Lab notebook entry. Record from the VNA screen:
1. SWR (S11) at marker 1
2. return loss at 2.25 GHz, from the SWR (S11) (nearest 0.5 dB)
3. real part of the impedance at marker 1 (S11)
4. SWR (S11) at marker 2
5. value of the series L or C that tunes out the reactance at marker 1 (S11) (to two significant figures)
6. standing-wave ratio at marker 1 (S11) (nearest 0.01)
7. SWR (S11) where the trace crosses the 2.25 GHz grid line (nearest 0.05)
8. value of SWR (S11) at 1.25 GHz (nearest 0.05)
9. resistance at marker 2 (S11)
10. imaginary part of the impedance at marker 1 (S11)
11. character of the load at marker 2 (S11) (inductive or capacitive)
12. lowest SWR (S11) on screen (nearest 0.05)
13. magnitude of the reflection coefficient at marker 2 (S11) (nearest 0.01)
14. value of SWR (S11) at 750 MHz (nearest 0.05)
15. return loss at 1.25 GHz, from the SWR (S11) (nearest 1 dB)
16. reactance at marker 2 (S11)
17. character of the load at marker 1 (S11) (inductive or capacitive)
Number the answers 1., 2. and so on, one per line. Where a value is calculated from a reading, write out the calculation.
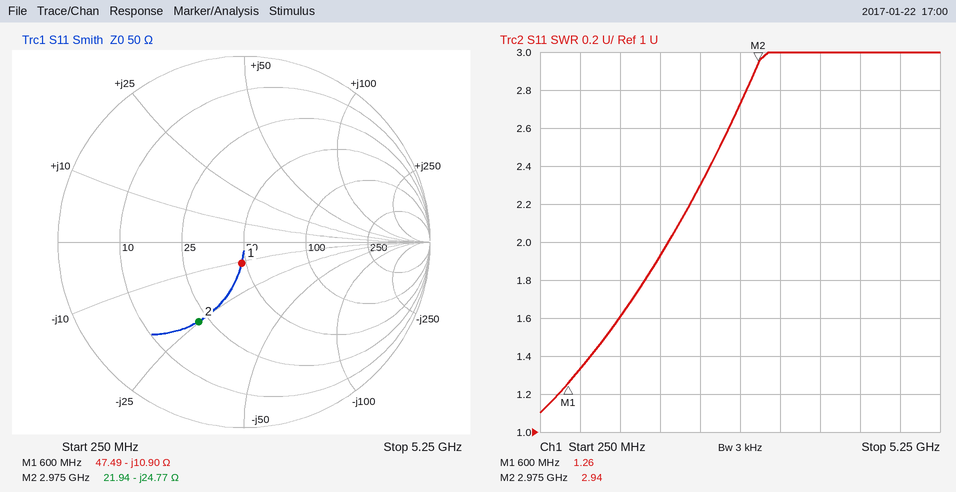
1. 1.26
2. −20 log10((2.3 − 1)/(2.3 + 1)) ≈ 8.09 dB, so 8.0 dB to the nearest 0.5 dB
3. 47.49 Ω
4. 2.94
5. L = 10.9 Ω/(2π × 600 MHz) ≈ 2.9 nH
6. 1.26
7. 2.30
8. 1.60
9. 21.94 Ω
10. -10.90 Ω
11. capacitive
12. 1.10
13. 0.49
14. 1.35
15. −20 log10((1.6 − 1)/(1.6 + 1)) ≈ 13 dB
16. -24.77 Ω
17. capacitive
